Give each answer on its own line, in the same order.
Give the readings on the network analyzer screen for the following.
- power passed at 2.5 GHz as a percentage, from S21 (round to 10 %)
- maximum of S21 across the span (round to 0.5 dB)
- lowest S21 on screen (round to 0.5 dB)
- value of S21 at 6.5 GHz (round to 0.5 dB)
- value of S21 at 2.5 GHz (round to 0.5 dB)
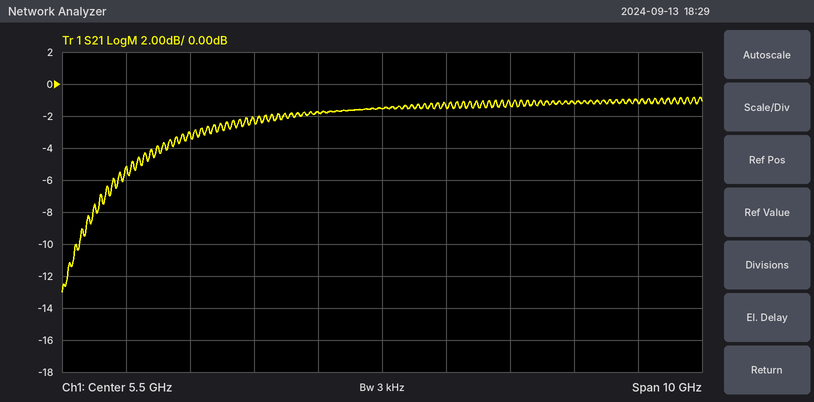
50 %
-1.0 dB
-13.0 dB
-1.5 dB
-3.0 dB
